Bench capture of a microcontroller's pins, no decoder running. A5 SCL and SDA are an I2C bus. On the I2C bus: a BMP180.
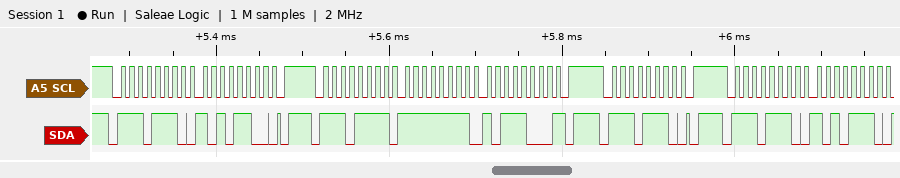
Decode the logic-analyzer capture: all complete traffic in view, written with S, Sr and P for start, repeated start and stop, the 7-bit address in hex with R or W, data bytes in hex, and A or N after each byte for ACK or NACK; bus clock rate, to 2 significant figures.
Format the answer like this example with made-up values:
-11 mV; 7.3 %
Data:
S 77W A AC A P S 77R A FF A B8 N P S 77W A P S 77W A AE A; 100 kHz
